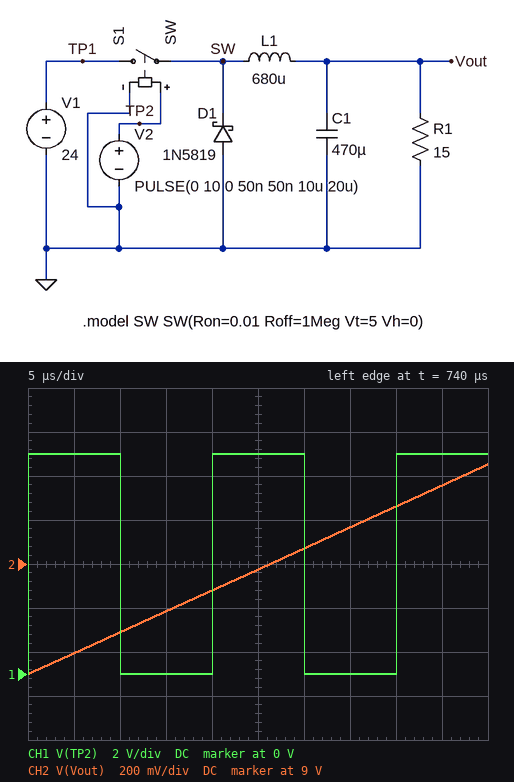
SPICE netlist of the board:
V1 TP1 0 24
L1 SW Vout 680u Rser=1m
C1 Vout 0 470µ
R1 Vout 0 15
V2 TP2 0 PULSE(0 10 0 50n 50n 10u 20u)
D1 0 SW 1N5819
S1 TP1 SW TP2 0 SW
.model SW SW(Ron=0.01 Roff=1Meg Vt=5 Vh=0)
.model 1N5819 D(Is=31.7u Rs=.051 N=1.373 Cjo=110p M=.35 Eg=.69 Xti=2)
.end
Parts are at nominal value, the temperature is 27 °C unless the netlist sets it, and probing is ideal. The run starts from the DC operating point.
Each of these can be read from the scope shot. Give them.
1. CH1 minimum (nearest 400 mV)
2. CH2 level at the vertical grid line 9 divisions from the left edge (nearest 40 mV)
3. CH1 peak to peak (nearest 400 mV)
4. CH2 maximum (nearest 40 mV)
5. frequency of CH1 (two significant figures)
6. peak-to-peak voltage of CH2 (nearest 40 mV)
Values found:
0 V
9.36 V
10.0 V
9.44 V
50 kHz
960 mV
